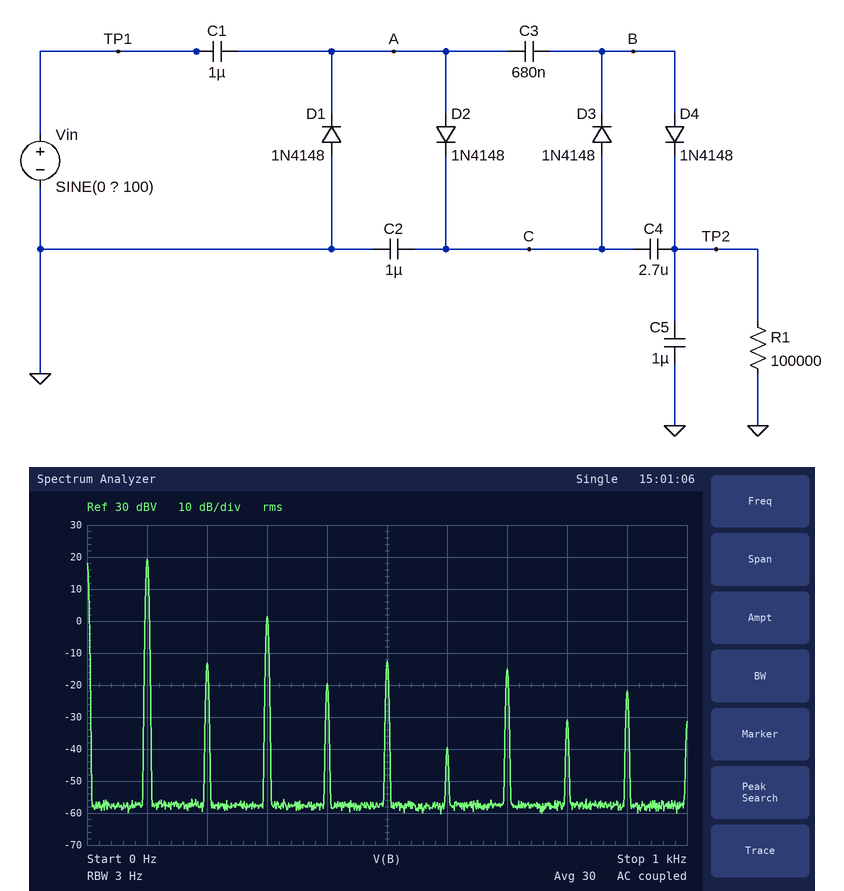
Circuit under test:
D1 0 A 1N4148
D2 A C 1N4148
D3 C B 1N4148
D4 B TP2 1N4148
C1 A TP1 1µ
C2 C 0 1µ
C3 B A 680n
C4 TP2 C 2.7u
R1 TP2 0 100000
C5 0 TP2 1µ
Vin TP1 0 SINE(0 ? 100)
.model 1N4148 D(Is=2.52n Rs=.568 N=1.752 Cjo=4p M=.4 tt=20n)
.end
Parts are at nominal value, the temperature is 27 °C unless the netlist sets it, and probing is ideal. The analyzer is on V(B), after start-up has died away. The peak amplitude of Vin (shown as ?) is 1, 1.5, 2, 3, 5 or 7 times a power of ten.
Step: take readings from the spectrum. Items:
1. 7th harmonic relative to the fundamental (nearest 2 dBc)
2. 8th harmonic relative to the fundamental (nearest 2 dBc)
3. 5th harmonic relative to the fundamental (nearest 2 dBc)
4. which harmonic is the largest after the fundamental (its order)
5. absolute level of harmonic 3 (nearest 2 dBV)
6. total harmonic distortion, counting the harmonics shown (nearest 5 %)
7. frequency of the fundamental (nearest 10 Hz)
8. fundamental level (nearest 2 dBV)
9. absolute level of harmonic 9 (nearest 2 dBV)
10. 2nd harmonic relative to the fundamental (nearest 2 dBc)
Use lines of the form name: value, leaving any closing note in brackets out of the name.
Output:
7th harmonic relative to the fundamental: -34 dBc
8th harmonic relative to the fundamental: -50 dBc
5th harmonic relative to the fundamental: -32 dBc
which harmonic is the largest after the fundamental: 3
absolute level of harmonic 3: 2 dBV
total harmonic distortion, counting the harmonics shown: 15 %
frequency of the fundamental: 100 Hz
fundamental level: 20 dBV
absolute level of harmonic 9: -22 dBV
2nd harmonic relative to the fundamental: -32 dBc
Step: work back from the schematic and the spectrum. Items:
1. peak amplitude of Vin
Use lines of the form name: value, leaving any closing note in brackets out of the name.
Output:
peak amplitude of Vin: 20 V
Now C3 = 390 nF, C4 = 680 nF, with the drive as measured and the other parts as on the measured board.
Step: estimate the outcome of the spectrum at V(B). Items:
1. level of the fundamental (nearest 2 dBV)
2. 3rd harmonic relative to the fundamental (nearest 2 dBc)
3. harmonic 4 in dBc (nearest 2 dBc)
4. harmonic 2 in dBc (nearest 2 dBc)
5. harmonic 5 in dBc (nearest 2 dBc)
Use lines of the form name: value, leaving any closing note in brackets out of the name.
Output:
level of the fundamental: 18 dBV
3rd harmonic relative to the fundamental: -16 dBc
harmonic 4 in dBc: -44 dBc
harmonic 2 in dBc: -36 dBc
harmonic 5 in dBc: -28 dBc
